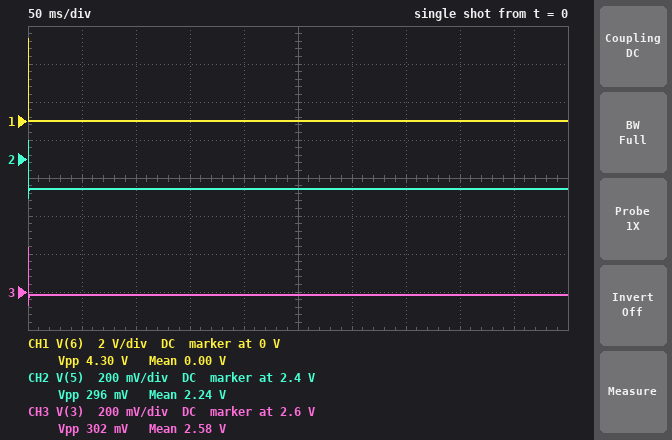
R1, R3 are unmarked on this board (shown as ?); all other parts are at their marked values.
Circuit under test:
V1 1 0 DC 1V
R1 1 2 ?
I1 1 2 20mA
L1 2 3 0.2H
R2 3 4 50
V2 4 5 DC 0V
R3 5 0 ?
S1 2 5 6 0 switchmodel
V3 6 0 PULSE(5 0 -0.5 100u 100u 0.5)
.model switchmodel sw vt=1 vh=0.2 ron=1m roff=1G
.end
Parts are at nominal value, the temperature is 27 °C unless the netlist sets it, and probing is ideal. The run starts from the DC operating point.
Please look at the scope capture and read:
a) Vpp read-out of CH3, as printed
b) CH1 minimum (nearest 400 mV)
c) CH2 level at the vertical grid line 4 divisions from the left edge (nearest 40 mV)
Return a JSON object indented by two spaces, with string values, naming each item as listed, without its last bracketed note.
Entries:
{
  "Vpp read-out of CH3, as printed": "302 mV",
  "CH1 minimum": "0 V",
  "CH2 level at the vertical grid line 4 divisions from the left edge": "2.24 V"
}
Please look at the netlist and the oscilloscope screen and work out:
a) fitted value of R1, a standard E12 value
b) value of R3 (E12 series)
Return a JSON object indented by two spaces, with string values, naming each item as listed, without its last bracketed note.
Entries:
{
  "fitted value of R1, a standard E12 value": "120 Ω",
  "value of R3": "330 Ω"
}
